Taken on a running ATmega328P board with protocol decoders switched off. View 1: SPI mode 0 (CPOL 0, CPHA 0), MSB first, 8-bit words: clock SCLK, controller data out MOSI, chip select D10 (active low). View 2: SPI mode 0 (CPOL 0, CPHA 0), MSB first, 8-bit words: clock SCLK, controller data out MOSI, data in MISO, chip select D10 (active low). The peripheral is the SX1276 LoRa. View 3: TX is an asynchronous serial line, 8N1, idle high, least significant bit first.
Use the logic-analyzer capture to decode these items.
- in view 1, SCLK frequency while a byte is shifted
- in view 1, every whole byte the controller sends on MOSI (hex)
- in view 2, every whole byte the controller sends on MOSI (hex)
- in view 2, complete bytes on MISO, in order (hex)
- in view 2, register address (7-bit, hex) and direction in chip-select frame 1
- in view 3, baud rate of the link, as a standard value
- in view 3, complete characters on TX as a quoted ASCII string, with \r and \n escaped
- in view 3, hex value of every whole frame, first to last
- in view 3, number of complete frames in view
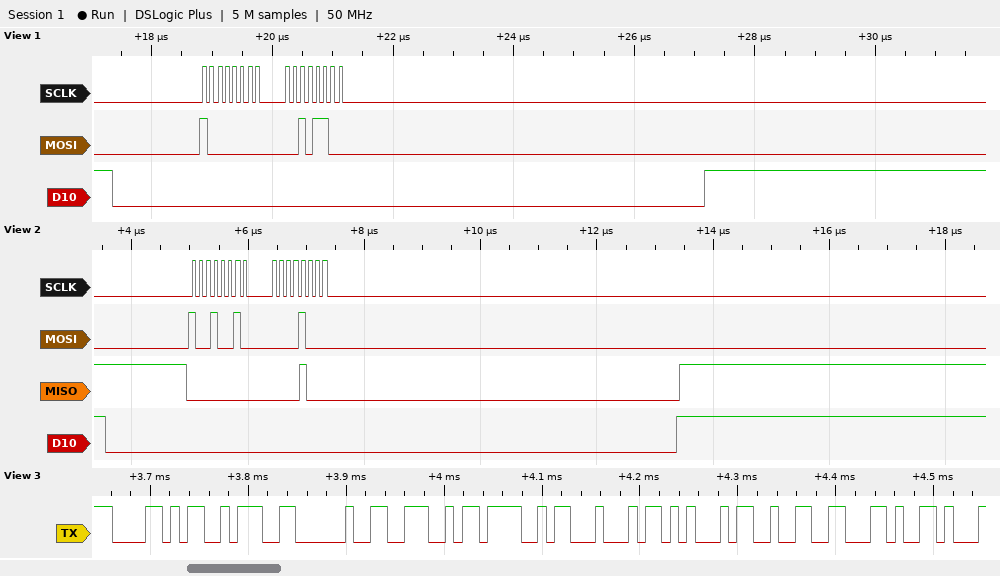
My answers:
8 MHz
80 2C
92 08
00 08
0x12 write
115200 baud
"X: NODE2,"
58 3A 20 4E 4F 44 45 32 2C
9
